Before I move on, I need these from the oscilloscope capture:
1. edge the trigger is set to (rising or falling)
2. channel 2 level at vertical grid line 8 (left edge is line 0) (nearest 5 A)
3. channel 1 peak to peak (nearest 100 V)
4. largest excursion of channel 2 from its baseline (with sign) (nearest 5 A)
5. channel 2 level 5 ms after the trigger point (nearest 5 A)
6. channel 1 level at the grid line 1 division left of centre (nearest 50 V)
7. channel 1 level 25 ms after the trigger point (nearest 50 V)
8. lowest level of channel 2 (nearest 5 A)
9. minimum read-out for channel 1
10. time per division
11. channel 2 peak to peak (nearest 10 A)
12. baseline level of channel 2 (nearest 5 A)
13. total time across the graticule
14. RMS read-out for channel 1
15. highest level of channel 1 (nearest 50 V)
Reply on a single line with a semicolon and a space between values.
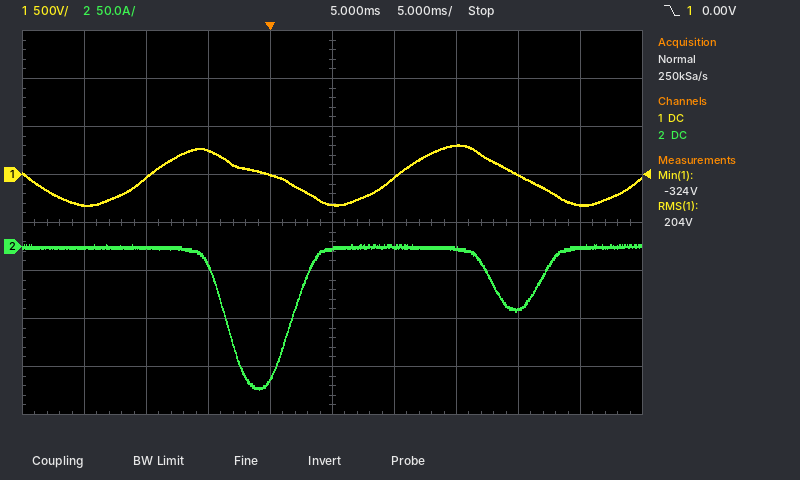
falling; -65 A; 600 V; -150 A; 0 A; 0 V; -300 V; -150 A; -324 V; 5 ms; 150 A; 0 A; 50 ms; 204 V; 300 V
